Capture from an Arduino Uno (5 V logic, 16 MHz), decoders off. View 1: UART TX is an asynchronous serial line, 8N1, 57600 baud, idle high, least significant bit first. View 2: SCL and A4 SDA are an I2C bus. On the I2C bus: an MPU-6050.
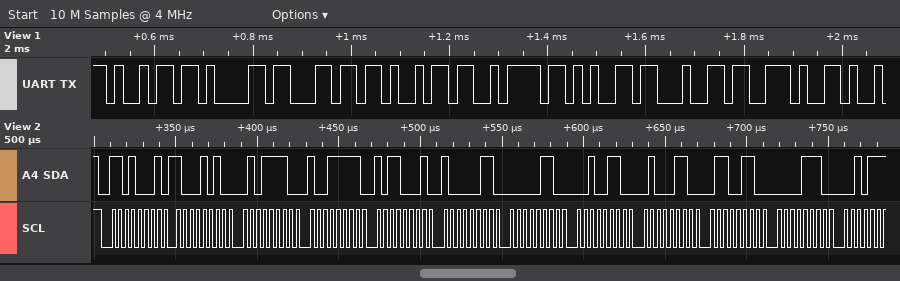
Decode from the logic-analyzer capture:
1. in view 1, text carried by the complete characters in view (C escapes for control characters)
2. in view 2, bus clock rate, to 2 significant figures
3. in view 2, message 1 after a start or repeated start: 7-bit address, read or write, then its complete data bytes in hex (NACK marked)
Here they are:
"ialized."
250 kHz
0x68 read: 8A 5E 9F B1 83 06 26 46 66 0E
